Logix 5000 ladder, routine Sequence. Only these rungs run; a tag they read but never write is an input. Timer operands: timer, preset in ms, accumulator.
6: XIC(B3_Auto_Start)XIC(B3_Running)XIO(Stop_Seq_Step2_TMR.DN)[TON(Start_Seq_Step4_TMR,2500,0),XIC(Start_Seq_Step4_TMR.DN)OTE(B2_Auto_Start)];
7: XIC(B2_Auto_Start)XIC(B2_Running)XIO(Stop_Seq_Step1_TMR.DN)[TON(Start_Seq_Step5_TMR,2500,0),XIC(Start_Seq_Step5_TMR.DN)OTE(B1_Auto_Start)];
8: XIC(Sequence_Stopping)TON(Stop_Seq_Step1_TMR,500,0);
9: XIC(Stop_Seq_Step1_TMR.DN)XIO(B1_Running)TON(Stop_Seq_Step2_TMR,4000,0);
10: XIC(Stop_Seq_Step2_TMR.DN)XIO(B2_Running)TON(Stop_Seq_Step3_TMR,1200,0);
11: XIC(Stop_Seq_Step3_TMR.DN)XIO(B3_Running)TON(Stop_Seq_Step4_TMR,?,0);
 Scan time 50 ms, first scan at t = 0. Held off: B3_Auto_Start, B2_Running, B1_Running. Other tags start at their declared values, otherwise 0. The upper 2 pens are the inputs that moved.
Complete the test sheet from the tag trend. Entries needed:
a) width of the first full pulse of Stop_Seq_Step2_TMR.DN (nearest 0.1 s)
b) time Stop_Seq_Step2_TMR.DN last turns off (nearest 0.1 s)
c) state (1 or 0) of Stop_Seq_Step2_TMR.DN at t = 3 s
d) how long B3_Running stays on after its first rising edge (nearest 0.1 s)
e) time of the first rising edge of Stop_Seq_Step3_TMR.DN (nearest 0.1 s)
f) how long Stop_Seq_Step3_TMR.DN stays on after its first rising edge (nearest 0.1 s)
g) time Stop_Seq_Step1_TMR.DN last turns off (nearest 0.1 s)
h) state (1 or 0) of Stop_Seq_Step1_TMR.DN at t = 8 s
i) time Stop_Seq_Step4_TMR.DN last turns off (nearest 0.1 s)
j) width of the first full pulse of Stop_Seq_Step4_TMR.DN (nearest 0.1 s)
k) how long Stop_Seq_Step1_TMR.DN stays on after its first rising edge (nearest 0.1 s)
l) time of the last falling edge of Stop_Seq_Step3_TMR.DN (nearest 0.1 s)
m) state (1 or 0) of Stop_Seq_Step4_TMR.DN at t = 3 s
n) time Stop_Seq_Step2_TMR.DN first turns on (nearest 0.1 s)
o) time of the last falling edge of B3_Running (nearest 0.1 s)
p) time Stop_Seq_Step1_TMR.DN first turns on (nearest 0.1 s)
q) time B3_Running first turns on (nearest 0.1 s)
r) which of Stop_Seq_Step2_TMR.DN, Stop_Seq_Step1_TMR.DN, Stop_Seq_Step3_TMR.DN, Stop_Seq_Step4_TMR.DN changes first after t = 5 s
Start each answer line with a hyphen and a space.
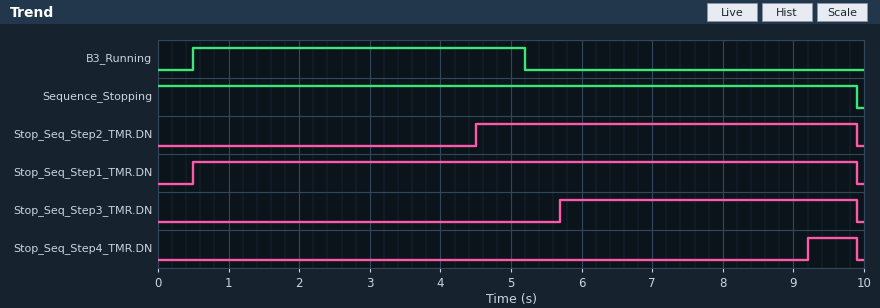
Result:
- 5.4 s
- 9.9 s
- 0
- 4.7 s
- 5.7 s
- 4.2 s
- 9.9 s
- 1
- 9.9 s
- 0.7 s
- 9.4 s
- 9.9 s
- 0
- 4.5 s
- 5.2 s
- 0.5 s
- 0.5 s
- Stop_Seq_Step3_TMR.DN
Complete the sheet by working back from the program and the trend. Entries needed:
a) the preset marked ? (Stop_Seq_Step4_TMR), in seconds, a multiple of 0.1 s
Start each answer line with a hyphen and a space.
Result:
- 3.5 s
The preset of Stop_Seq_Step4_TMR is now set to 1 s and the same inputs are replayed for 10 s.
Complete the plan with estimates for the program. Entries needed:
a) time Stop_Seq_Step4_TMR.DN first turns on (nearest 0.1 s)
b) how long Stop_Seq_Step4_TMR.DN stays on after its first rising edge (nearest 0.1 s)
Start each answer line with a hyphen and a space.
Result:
- 6.7 s
- 3.2 s
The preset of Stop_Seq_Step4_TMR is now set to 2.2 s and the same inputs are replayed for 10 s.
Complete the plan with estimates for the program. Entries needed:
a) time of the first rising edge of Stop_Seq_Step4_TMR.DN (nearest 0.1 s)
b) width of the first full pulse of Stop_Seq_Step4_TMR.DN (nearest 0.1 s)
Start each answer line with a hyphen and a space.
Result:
- 7.9 s
- 2.0 s
